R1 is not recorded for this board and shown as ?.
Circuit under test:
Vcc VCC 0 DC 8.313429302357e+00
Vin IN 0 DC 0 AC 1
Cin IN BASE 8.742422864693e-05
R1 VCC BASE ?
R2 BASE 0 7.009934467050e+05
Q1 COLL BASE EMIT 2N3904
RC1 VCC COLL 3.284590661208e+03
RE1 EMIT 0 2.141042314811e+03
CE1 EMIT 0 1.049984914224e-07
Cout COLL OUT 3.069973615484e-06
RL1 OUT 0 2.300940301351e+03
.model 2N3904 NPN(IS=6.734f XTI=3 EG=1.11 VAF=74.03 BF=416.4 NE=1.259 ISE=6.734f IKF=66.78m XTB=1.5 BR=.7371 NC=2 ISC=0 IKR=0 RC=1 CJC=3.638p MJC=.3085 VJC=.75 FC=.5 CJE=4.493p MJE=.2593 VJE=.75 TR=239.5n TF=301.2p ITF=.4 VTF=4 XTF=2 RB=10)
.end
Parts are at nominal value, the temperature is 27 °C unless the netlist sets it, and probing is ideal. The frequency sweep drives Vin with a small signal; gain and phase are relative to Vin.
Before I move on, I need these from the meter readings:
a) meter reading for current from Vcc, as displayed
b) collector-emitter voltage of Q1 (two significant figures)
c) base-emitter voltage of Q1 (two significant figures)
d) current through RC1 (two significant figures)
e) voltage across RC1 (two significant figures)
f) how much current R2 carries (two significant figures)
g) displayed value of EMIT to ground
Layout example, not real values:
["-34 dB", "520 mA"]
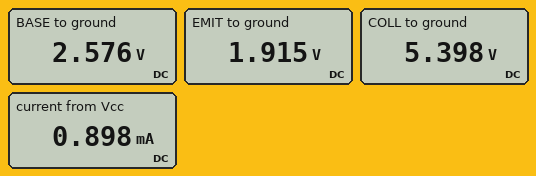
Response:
["0.898 mA", "3.5 V", "660 mV", "890 µA", "2.9 V", "3.7 µA", "1.915 V"]
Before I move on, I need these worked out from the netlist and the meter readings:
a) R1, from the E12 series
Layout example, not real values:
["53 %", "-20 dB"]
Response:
["560 kΩ"]
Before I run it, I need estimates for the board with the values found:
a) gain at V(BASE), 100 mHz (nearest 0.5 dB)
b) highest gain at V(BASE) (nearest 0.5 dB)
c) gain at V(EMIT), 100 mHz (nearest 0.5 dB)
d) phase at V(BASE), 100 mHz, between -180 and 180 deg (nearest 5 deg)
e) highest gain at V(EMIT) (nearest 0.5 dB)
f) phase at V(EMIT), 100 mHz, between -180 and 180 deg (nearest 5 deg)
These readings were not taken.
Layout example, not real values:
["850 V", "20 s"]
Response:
["0 dB", "0 dB", "0 dB", "5 deg", "0 dB", "5 deg"]
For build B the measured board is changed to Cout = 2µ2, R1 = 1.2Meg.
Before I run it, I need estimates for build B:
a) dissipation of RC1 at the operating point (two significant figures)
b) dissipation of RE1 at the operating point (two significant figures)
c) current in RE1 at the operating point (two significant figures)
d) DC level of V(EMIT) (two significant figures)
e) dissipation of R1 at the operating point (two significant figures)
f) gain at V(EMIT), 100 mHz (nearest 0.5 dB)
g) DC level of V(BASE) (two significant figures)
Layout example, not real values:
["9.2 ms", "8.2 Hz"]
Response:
["600 µW", "400 µW", "430 µA", "920 mV", "38 µW", "-0.5 dB", "1.6 V"]
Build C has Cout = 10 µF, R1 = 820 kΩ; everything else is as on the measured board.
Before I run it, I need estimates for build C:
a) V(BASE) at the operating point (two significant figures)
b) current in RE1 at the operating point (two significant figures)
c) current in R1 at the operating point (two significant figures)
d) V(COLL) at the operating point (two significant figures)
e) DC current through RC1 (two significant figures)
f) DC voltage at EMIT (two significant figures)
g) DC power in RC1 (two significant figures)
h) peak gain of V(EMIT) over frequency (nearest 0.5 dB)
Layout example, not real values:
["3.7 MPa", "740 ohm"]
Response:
["2.0 V", "640 µA", "7.7 µA", "6.2 V", "630 µA", "1.4 V", "1.3 mW", "0 dB"]
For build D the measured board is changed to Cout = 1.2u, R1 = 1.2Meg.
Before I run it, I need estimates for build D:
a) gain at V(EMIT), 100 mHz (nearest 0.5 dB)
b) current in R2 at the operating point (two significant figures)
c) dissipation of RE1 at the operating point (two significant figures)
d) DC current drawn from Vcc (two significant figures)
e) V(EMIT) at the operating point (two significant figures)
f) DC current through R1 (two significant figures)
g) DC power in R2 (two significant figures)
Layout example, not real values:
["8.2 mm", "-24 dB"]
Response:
["-0.5 dB", "2.2 µA", "400 µW", "430 µA", "920 mV", "5.6 µA", "3.5 µW"]
